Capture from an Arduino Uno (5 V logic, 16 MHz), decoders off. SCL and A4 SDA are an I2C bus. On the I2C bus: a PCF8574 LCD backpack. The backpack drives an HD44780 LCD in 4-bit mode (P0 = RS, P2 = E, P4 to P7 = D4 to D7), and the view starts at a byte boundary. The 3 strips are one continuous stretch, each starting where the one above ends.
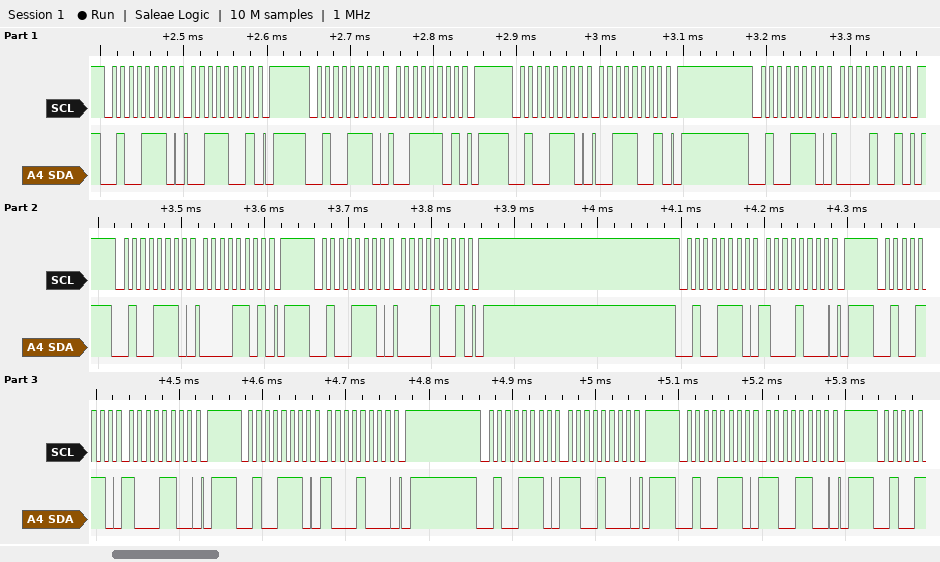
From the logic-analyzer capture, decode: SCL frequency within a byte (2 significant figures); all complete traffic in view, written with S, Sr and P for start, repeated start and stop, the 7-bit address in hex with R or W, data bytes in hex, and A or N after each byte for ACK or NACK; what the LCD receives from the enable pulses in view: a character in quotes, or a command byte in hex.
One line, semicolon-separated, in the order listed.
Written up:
100 kHz; S 27W A 39 A P S 27W A 3D A P S 27W A 39 A P S 27W A 09 A P S 27W A 0D A P S 27W A 09 A P S 27W A 88 A P S 27W A 8C A P S 27W A 88 A P S 27W A C8 A P S 27W A CC A P; '0'
